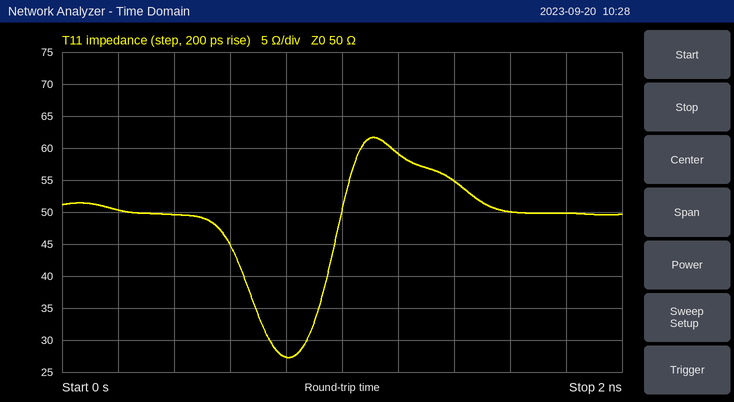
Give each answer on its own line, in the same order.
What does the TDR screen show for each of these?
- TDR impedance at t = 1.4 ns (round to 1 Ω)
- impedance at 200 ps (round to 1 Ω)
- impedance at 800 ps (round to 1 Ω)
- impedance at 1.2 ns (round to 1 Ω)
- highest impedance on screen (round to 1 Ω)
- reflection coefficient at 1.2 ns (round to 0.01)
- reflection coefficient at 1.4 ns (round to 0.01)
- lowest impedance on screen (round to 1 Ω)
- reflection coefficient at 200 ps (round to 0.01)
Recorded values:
55 Ω
50 Ω
27 Ω
59 Ω
62 Ω
+0.08
+0.05
27 Ω
0.00
